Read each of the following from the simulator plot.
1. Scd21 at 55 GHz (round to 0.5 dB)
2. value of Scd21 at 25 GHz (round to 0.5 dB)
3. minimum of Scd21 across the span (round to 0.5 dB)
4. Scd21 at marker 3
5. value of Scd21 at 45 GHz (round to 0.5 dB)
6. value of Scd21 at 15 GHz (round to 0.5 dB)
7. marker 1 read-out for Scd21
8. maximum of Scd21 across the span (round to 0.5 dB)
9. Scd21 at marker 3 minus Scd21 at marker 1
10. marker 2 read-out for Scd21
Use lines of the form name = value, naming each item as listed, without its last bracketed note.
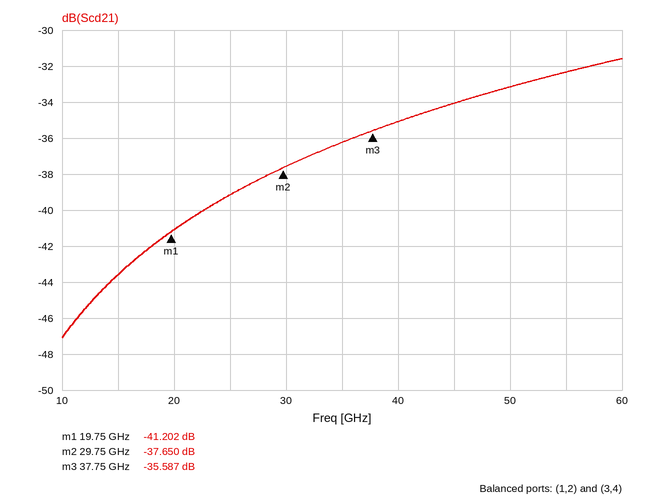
Scd21 at 55 GHz = -32.5 dB
value of Scd21 at 25 GHz = -39.0 dB
minimum of Scd21 across the span = -47.0 dB
Scd21 at marker 3 = -35.587 dB
value of Scd21 at 45 GHz = -34.0 dB
value of Scd21 at 15 GHz = -43.5 dB
marker 1 read-out for Scd21 = -41.202 dB
maximum of Scd21 across the span = -31.5 dB
Scd21 at marker 3 minus Scd21 at marker 1 = 5.615 dB
marker 2 read-out for Scd21 = -37.650 dB
